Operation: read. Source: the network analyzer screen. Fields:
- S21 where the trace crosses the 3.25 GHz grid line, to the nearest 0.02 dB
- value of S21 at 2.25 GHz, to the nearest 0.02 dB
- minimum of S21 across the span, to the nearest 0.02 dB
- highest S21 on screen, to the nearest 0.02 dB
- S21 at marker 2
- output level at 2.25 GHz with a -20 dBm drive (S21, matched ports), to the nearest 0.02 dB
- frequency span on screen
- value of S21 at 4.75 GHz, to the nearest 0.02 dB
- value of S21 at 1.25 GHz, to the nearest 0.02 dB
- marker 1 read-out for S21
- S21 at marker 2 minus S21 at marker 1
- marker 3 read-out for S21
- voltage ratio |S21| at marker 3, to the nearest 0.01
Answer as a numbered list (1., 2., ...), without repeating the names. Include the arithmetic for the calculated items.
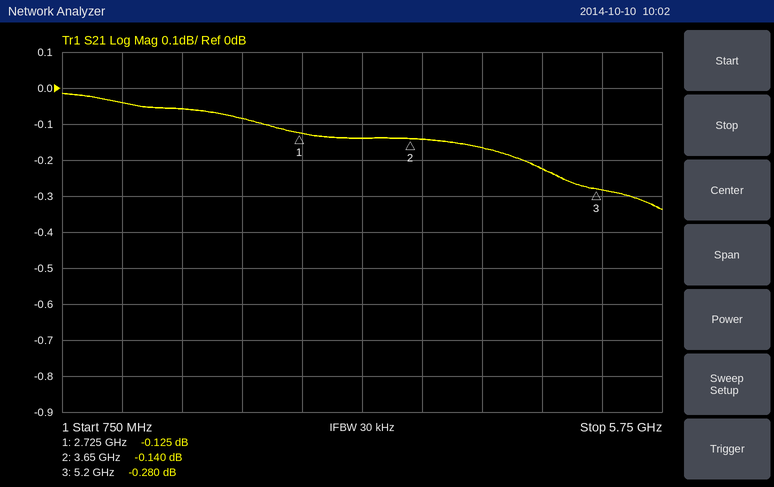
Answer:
1. -0.14 dB
2. -0.08 dB
3. -0.34 dB
4. -0.02 dB
5. -0.140 dB
6. -20 dBm + (-0.08 dB) = -20.08 dBm
7. 5 GHz
8. -0.22 dB
9. -0.04 dB
10. -0.125 dB
11. -0.14 − (-0.125) = -0.015 dB
12. -0.280 dB
13. 10^(-0.28/20) ≈ 0.97
